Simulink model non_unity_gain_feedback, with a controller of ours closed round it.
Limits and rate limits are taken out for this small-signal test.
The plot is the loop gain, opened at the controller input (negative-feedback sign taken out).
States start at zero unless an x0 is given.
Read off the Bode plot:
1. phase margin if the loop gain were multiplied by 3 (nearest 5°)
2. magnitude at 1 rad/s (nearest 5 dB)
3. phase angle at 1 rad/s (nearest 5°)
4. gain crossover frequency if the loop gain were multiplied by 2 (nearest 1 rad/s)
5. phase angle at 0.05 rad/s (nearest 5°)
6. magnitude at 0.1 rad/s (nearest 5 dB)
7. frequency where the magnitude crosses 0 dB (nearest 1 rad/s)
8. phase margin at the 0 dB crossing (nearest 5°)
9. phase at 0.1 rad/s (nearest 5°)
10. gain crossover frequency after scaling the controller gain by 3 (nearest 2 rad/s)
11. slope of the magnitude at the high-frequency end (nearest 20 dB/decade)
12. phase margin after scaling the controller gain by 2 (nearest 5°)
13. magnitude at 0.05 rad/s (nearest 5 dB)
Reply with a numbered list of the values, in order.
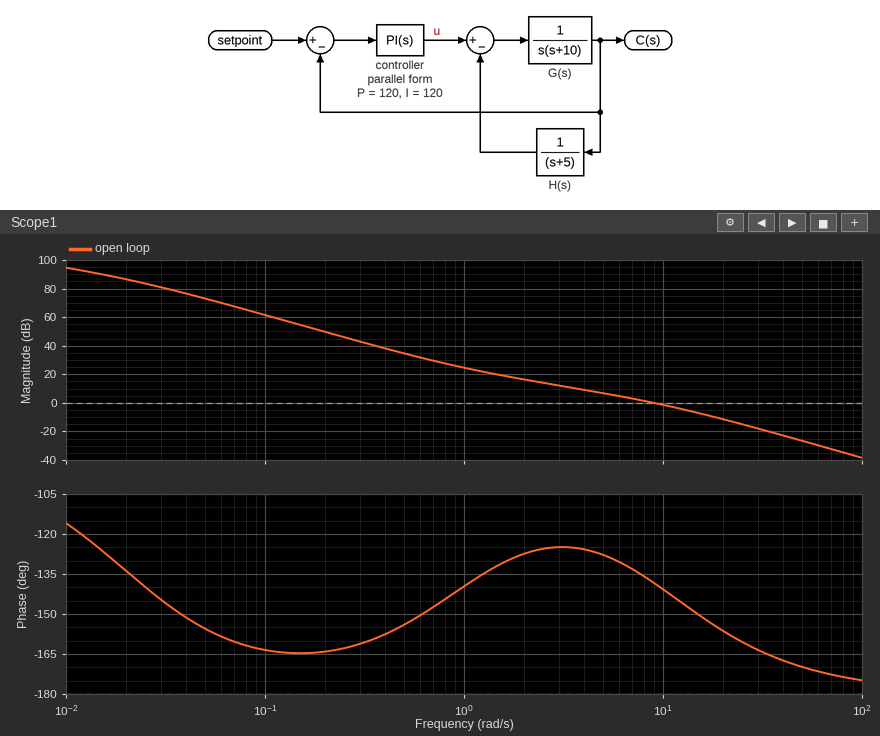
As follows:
1. 25°
2. 25 dB
3. -140°
4. 14 rad/s
5. -155°
6. 60 dB
7. 9 rad/s
8. 40°
9. -165°
10. 18 rad/s
11. -40 dB/decade
12. 30°
13. 75 dB
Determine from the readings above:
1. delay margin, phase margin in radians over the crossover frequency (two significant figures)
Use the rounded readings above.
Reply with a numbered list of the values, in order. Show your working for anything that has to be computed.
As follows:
1. 40 × π / 180 / 9 = 0.078 s
